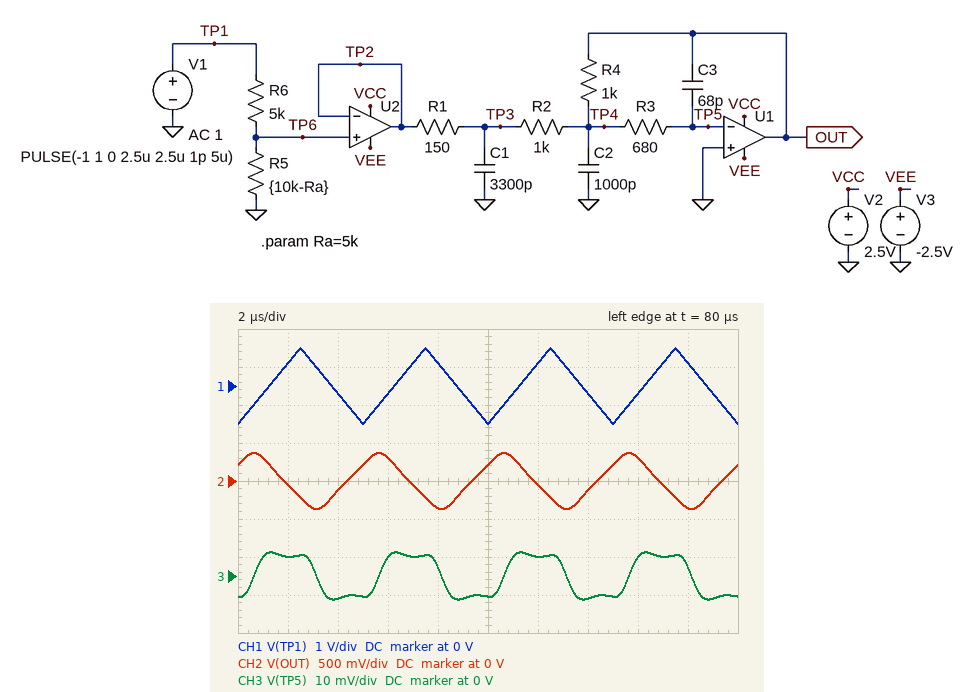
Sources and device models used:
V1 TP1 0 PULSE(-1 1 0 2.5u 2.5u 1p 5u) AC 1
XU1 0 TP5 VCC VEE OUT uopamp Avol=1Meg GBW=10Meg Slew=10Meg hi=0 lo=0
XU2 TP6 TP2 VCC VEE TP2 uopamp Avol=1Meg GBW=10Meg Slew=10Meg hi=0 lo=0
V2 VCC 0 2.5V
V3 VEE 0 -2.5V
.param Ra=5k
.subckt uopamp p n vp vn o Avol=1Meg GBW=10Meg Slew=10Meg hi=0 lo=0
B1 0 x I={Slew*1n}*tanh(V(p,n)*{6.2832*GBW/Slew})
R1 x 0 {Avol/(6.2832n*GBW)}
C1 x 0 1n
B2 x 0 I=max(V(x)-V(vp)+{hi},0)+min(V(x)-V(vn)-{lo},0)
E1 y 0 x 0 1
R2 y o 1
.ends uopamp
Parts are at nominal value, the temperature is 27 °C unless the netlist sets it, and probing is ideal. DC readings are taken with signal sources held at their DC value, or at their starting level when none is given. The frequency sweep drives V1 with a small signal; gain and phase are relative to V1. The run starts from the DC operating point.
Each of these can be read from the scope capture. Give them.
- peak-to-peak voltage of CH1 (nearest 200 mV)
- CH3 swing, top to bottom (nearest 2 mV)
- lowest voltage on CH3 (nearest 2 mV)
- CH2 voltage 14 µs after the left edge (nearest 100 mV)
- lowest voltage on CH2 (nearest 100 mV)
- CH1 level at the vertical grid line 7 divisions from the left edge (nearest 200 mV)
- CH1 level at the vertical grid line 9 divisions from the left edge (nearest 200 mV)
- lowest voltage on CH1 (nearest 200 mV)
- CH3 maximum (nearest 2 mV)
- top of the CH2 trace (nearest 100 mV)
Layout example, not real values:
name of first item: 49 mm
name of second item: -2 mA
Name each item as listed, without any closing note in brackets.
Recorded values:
peak-to-peak voltage of CH1: 2.0 V
CH3 swing, top to bottom: 12 mV
lowest voltage on CH3: -6 mV
CH2 voltage 14 µs after the left edge: -100 mV
lowest voltage on CH2: -400 mV
CH1 level at the vertical grid line 7 divisions from the left edge: -200 mV
CH1 level at the vertical grid line 9 divisions from the left edge: 600 mV
lowest voltage on CH1: -1.0 V
CH3 maximum: 6 mV
top of the CH2 trace: 400 mV
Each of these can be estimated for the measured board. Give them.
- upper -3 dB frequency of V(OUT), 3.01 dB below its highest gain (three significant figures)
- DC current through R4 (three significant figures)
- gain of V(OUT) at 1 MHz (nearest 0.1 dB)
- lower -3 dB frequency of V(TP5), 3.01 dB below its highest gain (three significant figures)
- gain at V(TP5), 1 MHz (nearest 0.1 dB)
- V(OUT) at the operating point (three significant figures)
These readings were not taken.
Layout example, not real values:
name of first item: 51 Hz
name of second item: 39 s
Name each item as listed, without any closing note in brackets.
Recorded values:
upper -3 dB frequency of V(OUT), 3.01 dB below its highest gain: 634 kHz
DC current through R4: 435 µA
gain of V(OUT) at 1 MHz: -21.9 dB
lower -3 dB frequency of V(TP5), 3.01 dB below its highest gain: 359 kHz
gain at V(TP5), 1 MHz: -41.9 dB
V(OUT) at the operating point: 435 mV
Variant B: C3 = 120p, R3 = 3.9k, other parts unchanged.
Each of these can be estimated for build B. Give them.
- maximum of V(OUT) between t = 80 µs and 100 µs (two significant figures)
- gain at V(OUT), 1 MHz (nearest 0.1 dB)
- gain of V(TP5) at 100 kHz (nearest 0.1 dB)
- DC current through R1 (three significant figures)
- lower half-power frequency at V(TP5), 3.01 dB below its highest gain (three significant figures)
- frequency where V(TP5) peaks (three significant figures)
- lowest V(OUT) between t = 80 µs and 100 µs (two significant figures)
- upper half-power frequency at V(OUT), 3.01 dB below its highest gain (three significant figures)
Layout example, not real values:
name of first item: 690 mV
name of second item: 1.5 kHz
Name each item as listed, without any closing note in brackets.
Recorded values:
maximum of V(OUT) between t = 80 µs and 100 µs: 240 mV
gain at V(OUT), 1 MHz: -42.3 dB
gain of V(TP5) at 100 kHz: -47.7 dB
DC current through R1: 435 µA
lower half-power frequency at V(TP5), 3.01 dB below its highest gain: 101 kHz
frequency where V(TP5) peaks: 197 kHz
lowest V(OUT) between t = 80 µs and 100 µs: -240 mV
upper half-power frequency at V(OUT), 3.01 dB below its highest gain: 191 kHz
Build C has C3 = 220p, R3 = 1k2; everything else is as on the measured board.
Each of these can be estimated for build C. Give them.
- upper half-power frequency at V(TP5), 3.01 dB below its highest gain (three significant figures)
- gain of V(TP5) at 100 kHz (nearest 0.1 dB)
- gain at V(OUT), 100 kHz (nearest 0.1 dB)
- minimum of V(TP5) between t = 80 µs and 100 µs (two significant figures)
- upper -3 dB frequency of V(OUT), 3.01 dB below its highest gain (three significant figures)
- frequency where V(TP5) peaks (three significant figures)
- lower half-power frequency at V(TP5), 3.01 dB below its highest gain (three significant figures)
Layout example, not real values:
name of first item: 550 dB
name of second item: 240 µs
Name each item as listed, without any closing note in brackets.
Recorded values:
upper half-power frequency at V(TP5), 3.01 dB below its highest gain: 428 kHz
gain of V(TP5) at 100 kHz: -47.5 dB
gain at V(OUT), 100 kHz: -7.5 dB
minimum of V(TP5) between t = 80 µs and 100 µs: -5.8 mV
upper -3 dB frequency of V(OUT), 3.01 dB below its highest gain: 245 kHz
frequency where V(TP5) peaks: 250 kHz
lower half-power frequency at V(TP5), 3.01 dB below its highest gain: 130 kHz
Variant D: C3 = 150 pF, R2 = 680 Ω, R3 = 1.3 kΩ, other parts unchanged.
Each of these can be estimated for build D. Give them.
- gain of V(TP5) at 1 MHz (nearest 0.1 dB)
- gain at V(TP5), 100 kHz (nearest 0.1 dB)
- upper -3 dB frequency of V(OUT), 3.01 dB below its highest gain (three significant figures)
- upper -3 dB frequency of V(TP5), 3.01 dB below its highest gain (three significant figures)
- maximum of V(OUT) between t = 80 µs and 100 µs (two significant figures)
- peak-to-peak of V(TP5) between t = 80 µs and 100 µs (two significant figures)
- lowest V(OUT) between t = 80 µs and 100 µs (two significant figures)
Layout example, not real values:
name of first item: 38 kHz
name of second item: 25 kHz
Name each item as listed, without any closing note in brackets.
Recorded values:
gain of V(TP5) at 1 MHz: -51.8 dB
gain at V(TP5), 100 kHz: -44.5 dB
upper -3 dB frequency of V(OUT), 3.01 dB below its highest gain: 285 kHz
upper -3 dB frequency of V(TP5), 3.01 dB below its highest gain: 474 kHz
maximum of V(OUT) between t = 80 µs and 100 µs: 440 mV
peak-to-peak of V(TP5) between t = 80 µs and 100 µs: 17 mV
lowest V(OUT) between t = 80 µs and 100 µs: -440 mV
